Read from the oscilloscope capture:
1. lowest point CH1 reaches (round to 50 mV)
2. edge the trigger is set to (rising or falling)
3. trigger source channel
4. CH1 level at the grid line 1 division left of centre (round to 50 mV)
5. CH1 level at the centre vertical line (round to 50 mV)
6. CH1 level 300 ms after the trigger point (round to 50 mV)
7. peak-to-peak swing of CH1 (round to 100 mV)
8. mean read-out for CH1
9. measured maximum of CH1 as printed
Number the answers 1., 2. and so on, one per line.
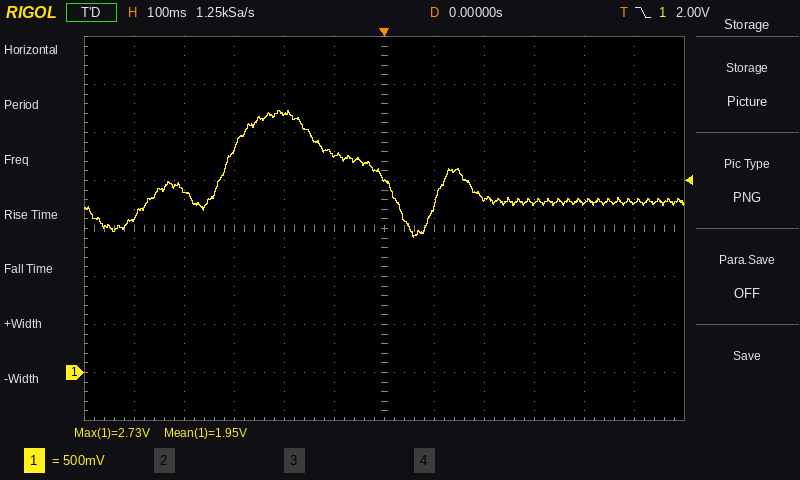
1. 1.40 V
2. falling
3. CH1
4. 2.25 V
5. 2.00 V
6. 1.75 V
7. 1.30 V
8. 1.95 V
9. 2.73 V
